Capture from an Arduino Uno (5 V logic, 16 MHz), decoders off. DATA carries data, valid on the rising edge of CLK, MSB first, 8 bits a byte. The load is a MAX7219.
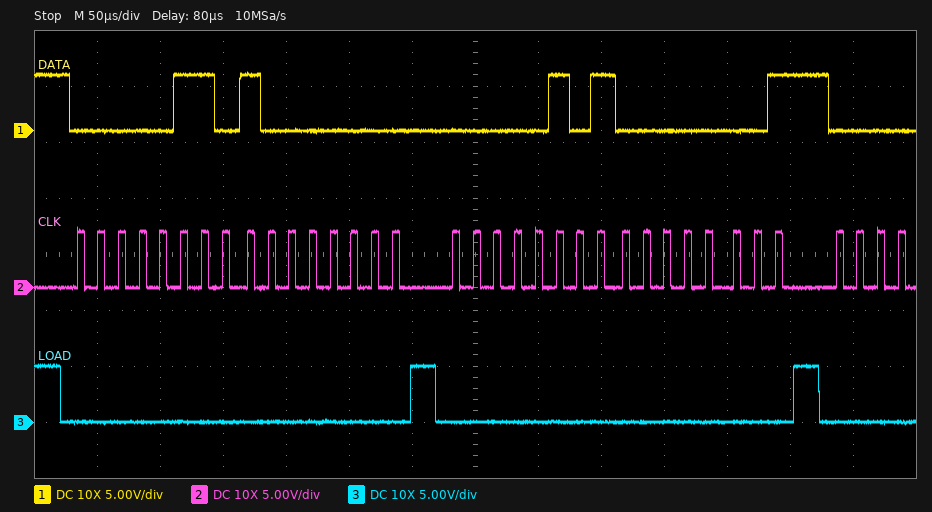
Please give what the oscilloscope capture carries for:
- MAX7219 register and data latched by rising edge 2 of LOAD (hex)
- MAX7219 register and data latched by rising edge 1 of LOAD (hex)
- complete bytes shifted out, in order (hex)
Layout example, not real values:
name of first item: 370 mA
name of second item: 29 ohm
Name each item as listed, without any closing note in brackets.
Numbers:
MAX7219 register and data latched by rising edge 2 of LOAD: register 0x5, data 0x01
MAX7219 register and data latched by rising edge 1 of LOAD: register 0x6, data 0x80
complete bytes shifted out, in order: 06 80 05 01
